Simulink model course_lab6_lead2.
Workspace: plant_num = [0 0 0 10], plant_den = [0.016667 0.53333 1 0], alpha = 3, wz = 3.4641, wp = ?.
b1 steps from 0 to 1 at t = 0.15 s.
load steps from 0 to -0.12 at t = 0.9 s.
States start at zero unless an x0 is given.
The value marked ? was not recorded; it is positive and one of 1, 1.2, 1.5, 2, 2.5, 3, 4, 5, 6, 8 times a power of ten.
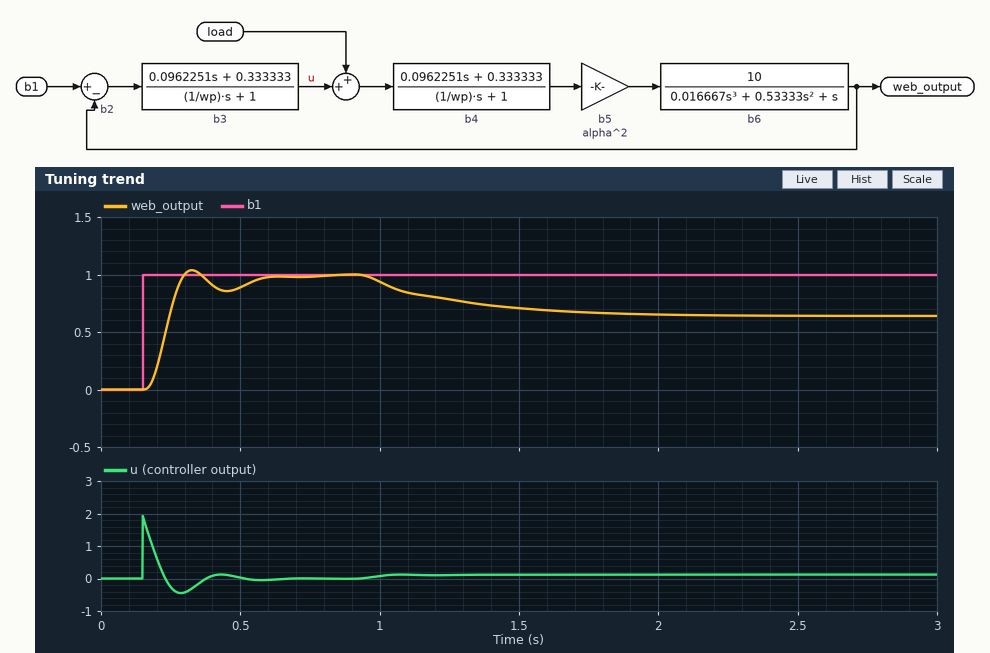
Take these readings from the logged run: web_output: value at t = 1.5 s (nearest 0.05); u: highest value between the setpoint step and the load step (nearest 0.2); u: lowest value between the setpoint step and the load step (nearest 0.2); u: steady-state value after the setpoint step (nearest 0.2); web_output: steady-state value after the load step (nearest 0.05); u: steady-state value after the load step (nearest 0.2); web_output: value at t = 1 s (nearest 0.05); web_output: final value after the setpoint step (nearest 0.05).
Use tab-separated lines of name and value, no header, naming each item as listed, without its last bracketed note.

web_output: value at t = 1.5 s	0.70
u: highest value between the setpoint step and the load step	2.0
u: lowest value between the setpoint step and the load step	-0.4
u: steady-state value after the setpoint step	0.0
web_output: steady-state value after the load step	0.65
u: steady-state value after the load step	0.2
web_output: value at t = 1 s	0.95
web_output: final value after the setpoint step	1.00
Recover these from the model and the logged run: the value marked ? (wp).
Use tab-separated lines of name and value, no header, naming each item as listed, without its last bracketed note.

the value marked ?	20
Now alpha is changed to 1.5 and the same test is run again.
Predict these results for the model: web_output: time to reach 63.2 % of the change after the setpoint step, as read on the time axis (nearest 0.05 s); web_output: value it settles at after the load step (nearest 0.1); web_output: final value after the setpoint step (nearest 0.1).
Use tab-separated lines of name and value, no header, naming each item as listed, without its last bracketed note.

web_output: time to reach 63.2 % of the change after the setpoint step, as read on the time axis	0.25 s
web_output: value it settles at after the load step	0.8
web_output: final value after the setpoint step	1.0
